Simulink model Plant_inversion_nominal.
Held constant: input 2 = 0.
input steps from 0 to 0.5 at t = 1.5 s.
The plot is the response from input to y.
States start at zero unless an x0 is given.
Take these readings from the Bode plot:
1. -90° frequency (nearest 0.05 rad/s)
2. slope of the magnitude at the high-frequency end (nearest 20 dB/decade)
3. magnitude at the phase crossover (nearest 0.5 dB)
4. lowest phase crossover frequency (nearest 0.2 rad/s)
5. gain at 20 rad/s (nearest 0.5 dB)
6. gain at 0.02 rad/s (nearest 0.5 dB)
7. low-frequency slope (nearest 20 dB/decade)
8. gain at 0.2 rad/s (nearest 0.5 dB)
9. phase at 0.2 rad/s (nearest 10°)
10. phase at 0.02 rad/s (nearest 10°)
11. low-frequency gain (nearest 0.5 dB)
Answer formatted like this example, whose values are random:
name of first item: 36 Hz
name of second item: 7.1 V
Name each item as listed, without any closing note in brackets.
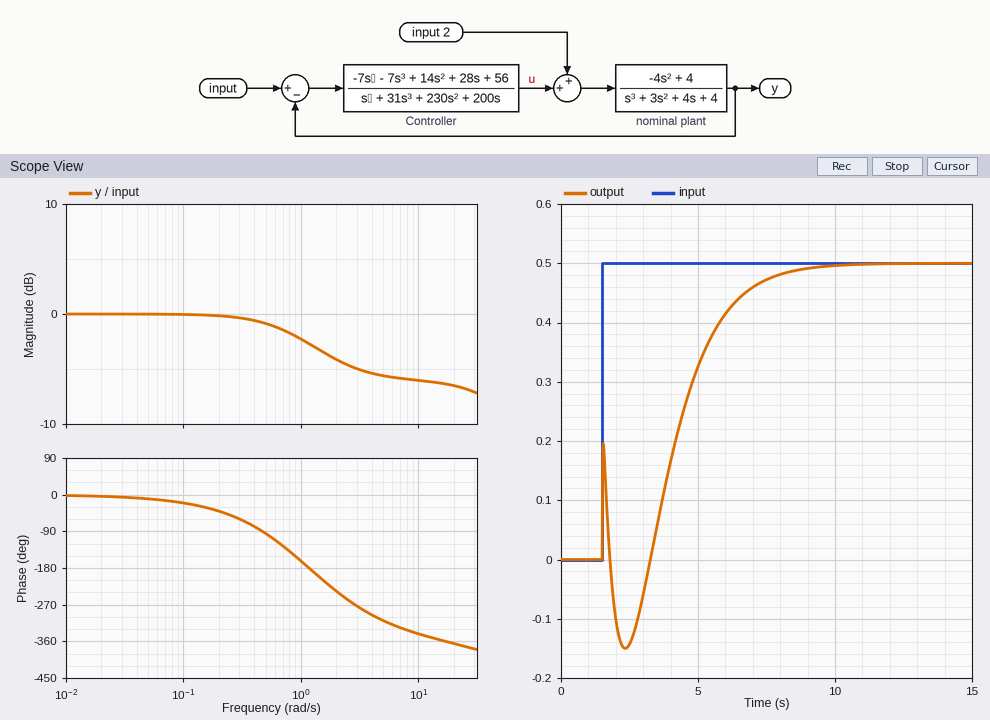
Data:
-90° frequency: 0.45 rad/s
slope of the magnitude at the high-frequency end: 0 dB/decade
magnitude at the phase crossover: -2.5 dB
lowest phase crossover frequency: 1.2 rad/s
gain at 20 rad/s: -6.5 dB
gain at 0.02 rad/s: 0.0 dB
low-frequency slope: 0 dB/decade
gain at 0.2 rad/s: 0.0 dB
phase at 0.2 rad/s: -40°
phase at 0.02 rad/s: 0°
low-frequency gain: 0.0 dB
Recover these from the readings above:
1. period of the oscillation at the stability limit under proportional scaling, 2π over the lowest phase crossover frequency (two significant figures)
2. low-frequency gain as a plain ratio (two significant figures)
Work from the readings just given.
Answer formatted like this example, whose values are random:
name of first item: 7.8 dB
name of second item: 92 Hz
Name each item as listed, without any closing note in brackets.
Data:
period of the oscillation at the stability limit under proportional scaling, 2π over the lowest phase crossover frequency: 5.2 s
low-frequency gain as a plain ratio: 1.0
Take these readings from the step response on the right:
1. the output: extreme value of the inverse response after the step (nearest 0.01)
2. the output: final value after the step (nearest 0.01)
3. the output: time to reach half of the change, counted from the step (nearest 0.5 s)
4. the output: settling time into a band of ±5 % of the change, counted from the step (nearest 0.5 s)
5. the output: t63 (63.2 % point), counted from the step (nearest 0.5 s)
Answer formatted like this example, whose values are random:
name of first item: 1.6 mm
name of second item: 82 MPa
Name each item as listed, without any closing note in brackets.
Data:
the output: extreme value of the inverse response after the step: -0.15
the output: final value after the step: 0.50
the output: time to reach half of the change, counted from the step: 3.0 s
the output: settling time into a band of ±5 % of the change, counted from the step: 6.0 s
the output: t63 (63.2 % point), counted from the step: 3.5 s
